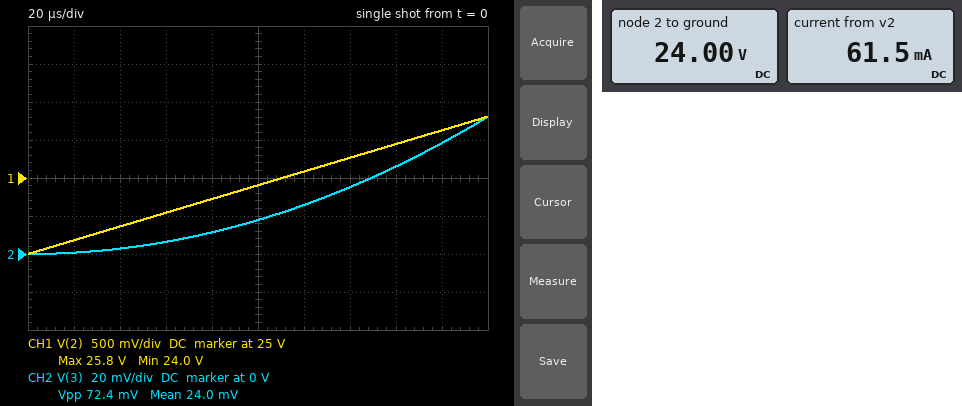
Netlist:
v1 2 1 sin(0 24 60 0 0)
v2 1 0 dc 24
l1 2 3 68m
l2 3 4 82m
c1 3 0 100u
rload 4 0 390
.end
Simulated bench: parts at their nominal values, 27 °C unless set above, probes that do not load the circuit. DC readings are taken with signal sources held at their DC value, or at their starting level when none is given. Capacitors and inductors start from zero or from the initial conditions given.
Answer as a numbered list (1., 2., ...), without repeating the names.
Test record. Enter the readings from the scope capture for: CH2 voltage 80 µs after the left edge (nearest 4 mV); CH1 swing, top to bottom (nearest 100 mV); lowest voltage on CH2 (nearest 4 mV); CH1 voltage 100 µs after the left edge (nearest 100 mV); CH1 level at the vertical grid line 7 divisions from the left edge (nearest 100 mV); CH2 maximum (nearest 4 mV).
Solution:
1. 12 mV
2. 1.8 V
3. 0 V
4. 24.9 V
5. 25.3 V
6. 72 mV
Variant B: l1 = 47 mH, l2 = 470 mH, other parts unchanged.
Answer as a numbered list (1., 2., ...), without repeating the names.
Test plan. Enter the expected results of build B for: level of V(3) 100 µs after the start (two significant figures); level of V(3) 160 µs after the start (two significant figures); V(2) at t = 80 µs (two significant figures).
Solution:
1. 26 mV
2. 67 mV
3. 25 V
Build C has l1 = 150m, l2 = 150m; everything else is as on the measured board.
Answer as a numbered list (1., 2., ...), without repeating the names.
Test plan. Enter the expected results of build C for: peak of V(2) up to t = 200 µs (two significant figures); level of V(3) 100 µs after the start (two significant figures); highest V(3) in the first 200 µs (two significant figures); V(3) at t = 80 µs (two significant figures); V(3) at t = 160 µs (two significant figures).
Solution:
1. 26 V
2. 8.1 mV
3. 33 mV
4. 5.2 mV
5. 21 mV
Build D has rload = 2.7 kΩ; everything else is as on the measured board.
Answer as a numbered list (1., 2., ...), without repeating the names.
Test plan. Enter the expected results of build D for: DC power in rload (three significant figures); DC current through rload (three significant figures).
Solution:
1. 213 mW
2. 8.89 mA
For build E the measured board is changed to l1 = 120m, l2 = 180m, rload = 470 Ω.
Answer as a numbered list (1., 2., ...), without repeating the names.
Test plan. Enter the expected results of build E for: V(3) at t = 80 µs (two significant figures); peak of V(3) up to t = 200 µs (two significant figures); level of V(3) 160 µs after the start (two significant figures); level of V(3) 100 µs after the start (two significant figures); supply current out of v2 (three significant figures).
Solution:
1. 6.5 mV
2. 41 mV
3. 26 mV
4. 10 mV
5. 51.1 mA
